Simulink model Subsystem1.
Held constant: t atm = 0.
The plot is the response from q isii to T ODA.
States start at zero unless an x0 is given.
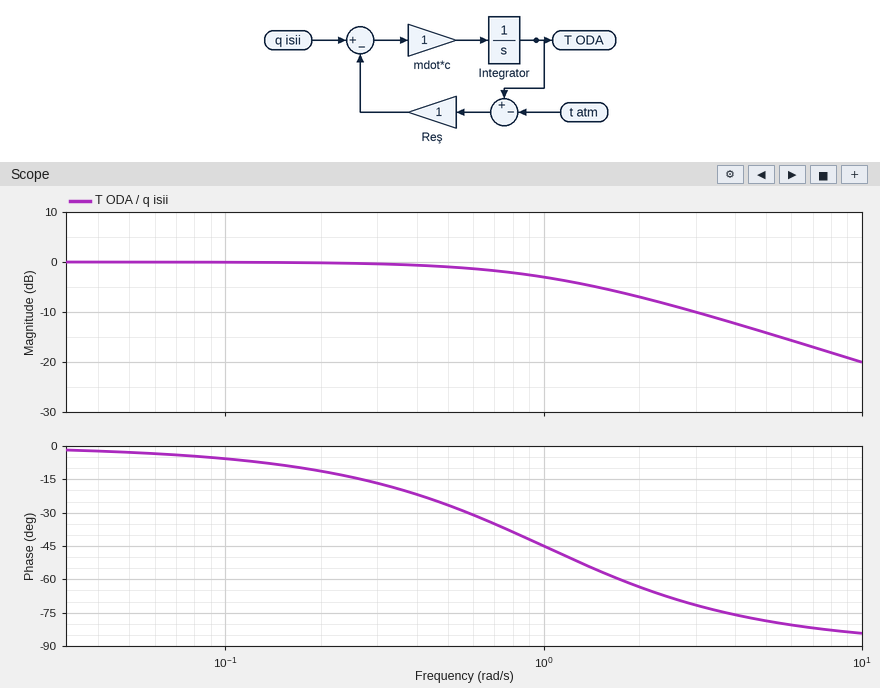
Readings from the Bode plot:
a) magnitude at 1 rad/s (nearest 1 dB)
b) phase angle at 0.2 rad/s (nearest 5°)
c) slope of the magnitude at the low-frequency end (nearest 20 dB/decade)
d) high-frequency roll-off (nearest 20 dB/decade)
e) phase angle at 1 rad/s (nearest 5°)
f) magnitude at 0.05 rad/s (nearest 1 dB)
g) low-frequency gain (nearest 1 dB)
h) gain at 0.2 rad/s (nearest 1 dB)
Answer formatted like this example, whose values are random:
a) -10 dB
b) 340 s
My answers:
a) -3 dB
b) -10°
c) 0 dB/decade
d) -20 dB/decade
e) -45°
f) 0 dB
g) 0 dB
h) 0 dB
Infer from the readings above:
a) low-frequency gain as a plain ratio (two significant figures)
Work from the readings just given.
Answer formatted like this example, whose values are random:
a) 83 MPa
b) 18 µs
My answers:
a) 1.0
